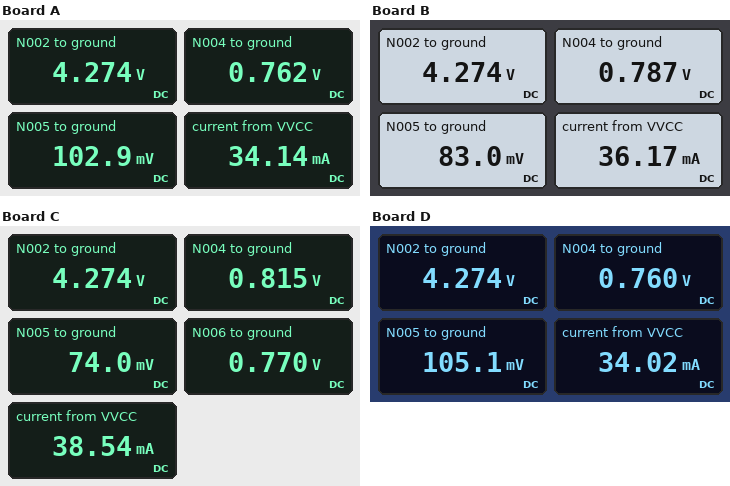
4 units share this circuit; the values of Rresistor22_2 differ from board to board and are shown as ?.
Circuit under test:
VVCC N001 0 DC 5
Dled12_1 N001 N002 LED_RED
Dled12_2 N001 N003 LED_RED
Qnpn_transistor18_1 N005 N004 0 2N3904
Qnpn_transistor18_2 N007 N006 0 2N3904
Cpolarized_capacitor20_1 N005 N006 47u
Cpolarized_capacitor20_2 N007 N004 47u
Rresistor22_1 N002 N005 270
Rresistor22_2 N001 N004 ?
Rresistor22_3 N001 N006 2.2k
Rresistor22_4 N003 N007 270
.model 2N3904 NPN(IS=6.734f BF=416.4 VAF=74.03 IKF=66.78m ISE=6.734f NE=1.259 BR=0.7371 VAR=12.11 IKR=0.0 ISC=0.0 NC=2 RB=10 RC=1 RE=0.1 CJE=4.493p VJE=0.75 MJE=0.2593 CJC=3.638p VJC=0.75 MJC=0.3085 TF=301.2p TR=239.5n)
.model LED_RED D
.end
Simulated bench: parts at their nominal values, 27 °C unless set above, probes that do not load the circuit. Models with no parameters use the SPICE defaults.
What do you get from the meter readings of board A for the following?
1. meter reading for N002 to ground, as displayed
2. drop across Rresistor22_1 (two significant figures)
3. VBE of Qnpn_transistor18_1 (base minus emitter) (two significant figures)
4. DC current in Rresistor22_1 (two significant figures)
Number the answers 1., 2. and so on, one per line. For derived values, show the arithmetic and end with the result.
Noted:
1. 4.274 V
2. 4.274 V - 102.9 mV = 4.2 V
3. 762 mV = 760 mV
4. (4.274 V - 102.9 mV) / 270 Ω = 15 mA
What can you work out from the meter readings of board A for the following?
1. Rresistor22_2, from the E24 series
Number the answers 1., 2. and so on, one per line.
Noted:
1. 3.3 kΩ
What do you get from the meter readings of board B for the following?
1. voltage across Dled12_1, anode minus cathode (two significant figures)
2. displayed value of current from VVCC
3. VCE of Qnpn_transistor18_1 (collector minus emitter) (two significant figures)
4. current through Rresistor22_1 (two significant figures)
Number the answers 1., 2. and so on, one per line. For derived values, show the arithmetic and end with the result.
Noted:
1. 5 V - 4.274 V = 730 mV
2. 36.17 mA
3. 83 mV = 83 mV
4. (4.274 V - 83 mV) / 270 Ω = 16 mA
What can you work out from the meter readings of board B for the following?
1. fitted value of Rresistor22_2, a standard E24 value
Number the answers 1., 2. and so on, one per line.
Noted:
1. 1.3 kΩ
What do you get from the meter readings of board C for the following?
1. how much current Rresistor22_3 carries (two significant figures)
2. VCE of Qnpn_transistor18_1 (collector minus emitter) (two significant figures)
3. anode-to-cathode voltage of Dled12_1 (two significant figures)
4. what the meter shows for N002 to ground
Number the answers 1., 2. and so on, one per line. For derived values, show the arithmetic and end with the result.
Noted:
1. (5 V - 770 mV) / 2.2 kΩ = 1.9 mA
2. 74 mV = 74 mV
3. 5 V - 4.274 V = 730 mV
4. 4.274 V
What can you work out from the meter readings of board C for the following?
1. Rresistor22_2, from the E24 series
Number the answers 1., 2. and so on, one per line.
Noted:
1. 750 Ω
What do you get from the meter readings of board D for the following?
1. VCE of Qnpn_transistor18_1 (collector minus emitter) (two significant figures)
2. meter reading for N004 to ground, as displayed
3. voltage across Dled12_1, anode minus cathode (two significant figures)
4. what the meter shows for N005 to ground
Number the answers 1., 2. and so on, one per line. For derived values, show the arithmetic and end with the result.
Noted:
1. 105.1 mV = 110 mV
2. 0.760 V
3. 5 V - 4.274 V = 730 mV
4. 105.1 mV
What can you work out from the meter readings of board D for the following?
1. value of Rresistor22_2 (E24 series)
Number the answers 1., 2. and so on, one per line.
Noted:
1. 3.6 kΩ
